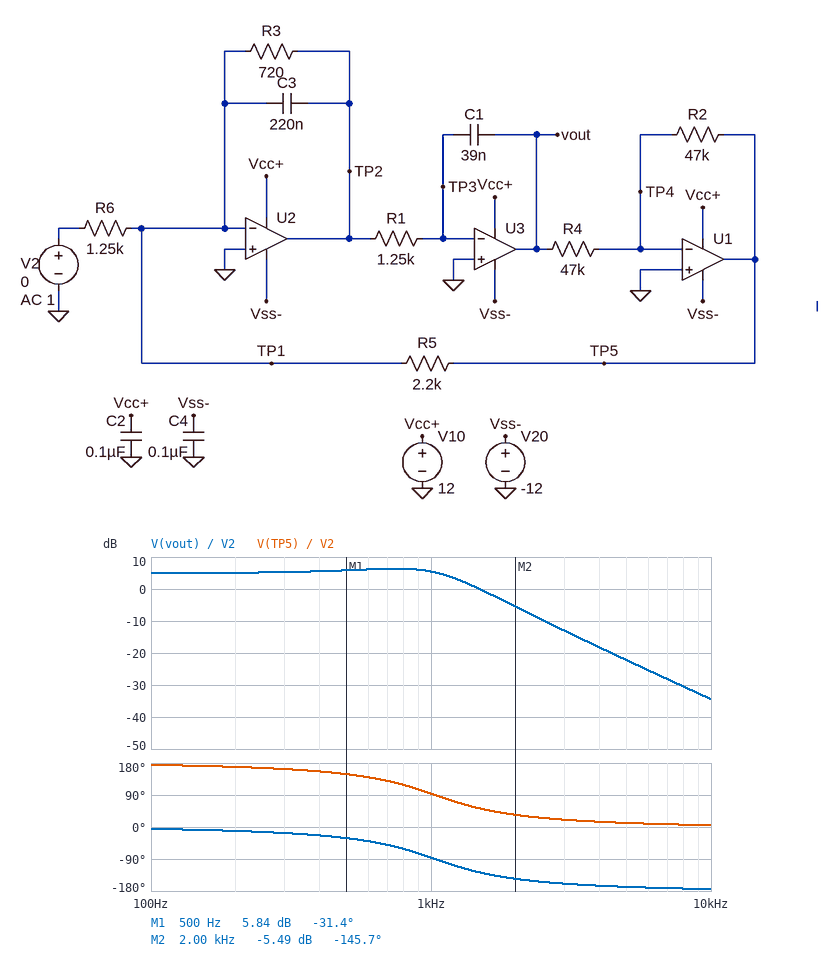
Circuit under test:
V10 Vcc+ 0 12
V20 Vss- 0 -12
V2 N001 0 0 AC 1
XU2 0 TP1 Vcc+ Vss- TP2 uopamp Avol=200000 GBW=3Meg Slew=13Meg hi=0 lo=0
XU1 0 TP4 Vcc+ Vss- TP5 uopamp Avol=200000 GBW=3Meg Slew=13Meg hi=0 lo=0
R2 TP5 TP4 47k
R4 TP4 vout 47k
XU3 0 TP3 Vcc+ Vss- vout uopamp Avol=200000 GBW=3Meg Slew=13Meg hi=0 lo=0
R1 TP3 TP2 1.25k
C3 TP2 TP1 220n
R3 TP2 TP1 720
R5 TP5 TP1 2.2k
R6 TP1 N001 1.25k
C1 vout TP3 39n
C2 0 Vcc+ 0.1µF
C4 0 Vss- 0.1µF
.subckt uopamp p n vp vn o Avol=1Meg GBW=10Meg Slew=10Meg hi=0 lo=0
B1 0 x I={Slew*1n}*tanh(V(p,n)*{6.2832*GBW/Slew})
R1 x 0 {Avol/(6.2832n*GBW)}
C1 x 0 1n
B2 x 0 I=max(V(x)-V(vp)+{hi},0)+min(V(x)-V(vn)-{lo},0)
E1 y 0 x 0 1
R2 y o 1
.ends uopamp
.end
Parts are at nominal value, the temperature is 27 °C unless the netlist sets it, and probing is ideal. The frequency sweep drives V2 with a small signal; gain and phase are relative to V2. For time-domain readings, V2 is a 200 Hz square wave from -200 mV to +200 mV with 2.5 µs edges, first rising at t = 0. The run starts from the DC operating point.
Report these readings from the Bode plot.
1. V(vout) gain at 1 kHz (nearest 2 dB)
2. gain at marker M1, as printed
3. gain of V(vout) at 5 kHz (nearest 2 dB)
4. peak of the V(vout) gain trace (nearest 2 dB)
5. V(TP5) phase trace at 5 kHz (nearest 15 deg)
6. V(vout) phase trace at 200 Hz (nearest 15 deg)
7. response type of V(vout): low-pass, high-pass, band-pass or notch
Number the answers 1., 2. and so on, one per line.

1. 6 dB
2. 5.84 dB
3. -22 dB
4. 6 dB
5. 15 deg
6. -15 deg
7. low-pass
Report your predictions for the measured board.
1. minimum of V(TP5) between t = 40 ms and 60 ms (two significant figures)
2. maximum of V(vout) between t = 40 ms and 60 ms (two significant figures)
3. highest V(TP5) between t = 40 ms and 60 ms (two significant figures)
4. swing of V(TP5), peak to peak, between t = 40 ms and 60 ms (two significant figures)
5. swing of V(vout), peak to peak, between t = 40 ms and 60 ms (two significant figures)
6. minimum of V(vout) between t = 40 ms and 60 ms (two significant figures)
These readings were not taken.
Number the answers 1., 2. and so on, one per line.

1. -480 mV
2. 480 mV
3. 480 mV
4. 950 mV
5. 950 mV
6. -480 mV
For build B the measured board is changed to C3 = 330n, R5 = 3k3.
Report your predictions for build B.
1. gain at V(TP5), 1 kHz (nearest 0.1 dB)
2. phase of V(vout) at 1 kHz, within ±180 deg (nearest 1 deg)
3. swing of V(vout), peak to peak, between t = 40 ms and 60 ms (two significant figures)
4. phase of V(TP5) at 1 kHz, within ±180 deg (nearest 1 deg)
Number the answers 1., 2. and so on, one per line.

1. 3.4 dB
2. -128 deg
3. 1.4 V
4. 52 deg
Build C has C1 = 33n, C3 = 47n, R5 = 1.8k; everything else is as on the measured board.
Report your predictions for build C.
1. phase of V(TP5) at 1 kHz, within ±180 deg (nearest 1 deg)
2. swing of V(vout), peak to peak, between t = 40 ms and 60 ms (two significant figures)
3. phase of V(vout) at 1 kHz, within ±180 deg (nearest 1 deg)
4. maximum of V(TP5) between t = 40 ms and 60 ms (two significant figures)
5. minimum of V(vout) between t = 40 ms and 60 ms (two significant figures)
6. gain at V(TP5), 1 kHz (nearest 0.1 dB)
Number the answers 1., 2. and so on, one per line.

1. 143 deg
2. 580 mV
3. -37 deg
4. 290 mV
5. -290 mV
6. 2.5 dB
